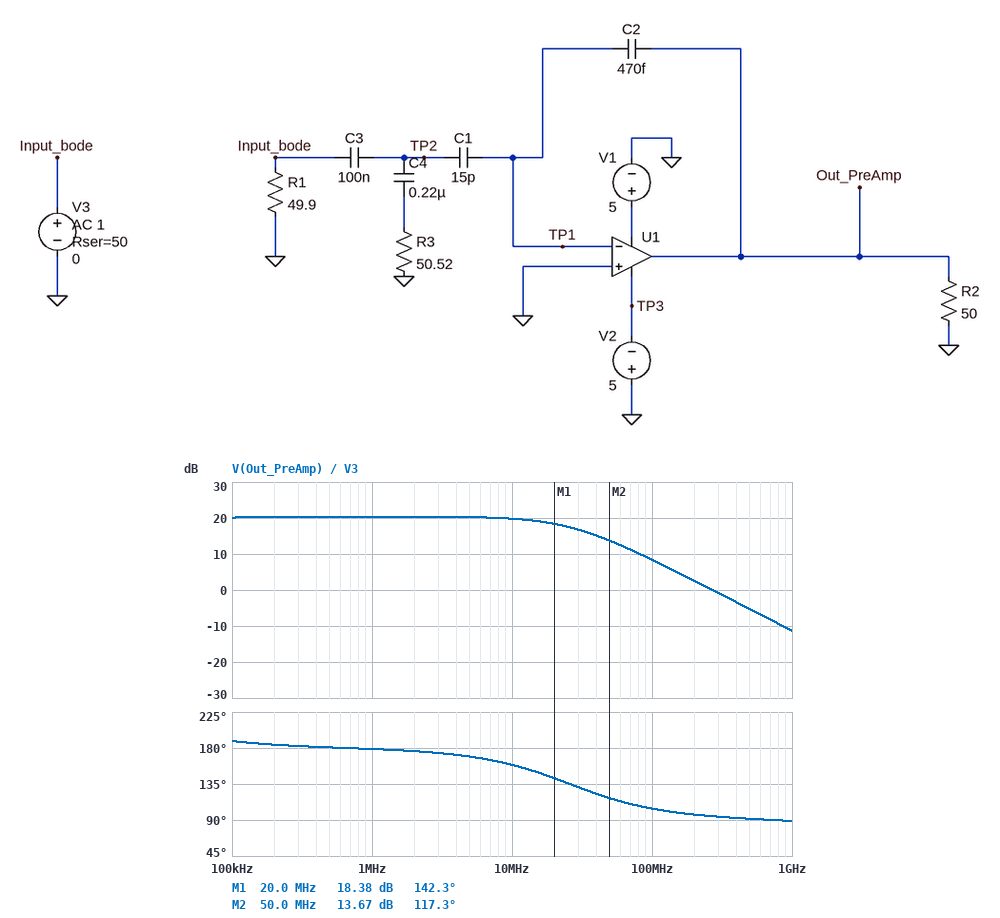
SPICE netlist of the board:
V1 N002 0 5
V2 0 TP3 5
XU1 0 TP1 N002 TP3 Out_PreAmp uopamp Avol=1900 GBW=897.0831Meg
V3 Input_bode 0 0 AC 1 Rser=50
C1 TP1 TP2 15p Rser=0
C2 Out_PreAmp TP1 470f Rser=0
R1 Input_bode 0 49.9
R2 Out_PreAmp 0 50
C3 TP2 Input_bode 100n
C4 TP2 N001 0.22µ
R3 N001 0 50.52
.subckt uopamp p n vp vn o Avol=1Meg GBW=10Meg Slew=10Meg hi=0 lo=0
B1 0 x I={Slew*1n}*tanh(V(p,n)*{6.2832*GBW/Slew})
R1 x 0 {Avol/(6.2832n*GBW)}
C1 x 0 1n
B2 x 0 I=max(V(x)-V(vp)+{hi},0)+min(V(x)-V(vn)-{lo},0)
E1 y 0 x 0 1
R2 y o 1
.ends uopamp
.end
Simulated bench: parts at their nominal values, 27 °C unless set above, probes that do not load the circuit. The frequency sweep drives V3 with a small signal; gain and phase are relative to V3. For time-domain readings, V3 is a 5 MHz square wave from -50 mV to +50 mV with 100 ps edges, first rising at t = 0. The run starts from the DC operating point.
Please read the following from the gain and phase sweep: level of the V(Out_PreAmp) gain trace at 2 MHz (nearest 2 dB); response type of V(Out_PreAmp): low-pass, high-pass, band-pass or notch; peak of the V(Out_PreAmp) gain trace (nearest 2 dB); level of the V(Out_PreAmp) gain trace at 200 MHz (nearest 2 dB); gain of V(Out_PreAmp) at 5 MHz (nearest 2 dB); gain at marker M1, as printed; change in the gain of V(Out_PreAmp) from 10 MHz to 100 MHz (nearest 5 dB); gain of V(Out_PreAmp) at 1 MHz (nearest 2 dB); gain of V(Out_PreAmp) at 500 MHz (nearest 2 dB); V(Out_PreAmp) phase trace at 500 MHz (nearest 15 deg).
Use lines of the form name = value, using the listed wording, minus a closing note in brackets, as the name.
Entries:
level of the V(Out_PreAmp) gain trace at 2 MHz = 20 dB
response type of V(Out_PreAmp): low-pass, high-pass, band-pass or notch = low-pass
peak of the V(Out_PreAmp) gain trace = 20 dB
level of the V(Out_PreAmp) gain trace at 200 MHz = 2 dB
gain of V(Out_PreAmp) at 5 MHz = 20 dB
gain at marker M1, as printed = 18.38 dB
change in the gain of V(Out_PreAmp) from 10 MHz to 100 MHz = -10 dB
gain of V(Out_PreAmp) at 1 MHz = 20 dB
gain of V(Out_PreAmp) at 500 MHz = -6 dB
V(Out_PreAmp) phase trace at 500 MHz = 90 deg
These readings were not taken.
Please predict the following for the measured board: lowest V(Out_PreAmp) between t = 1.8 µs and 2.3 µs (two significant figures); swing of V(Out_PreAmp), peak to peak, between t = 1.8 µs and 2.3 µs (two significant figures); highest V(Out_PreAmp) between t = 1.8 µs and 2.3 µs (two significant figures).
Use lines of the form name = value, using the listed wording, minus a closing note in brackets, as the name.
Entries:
lowest V(Out_PreAmp) between t = 1.8 µs and 2.3 µs = -790 mV
swing of V(Out_PreAmp), peak to peak, between t = 1.8 µs and 2.3 µs = 880 mV
highest V(Out_PreAmp) between t = 1.8 µs and 2.3 µs = 94 mV
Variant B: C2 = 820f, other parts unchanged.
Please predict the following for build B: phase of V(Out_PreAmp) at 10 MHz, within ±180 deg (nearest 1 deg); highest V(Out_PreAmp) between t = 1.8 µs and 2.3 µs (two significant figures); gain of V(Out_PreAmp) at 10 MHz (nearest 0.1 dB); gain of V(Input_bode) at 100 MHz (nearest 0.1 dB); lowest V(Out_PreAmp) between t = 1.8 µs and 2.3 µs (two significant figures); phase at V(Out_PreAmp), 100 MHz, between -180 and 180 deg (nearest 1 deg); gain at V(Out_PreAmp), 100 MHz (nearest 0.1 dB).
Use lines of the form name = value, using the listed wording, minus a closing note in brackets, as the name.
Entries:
phase of V(Out_PreAmp) at 10 MHz, within ±180 deg = 167 deg
highest V(Out_PreAmp) between t = 1.8 µs and 2.3 µs = 55 mV
gain of V(Out_PreAmp) at 10 MHz = 15.4 dB
gain of V(Input_bode) at 100 MHz = -10.0 dB
lowest V(Out_PreAmp) between t = 1.8 µs and 2.3 µs = -550 mV
phase at V(Out_PreAmp), 100 MHz, between -180 and 180 deg = 113 deg
gain at V(Out_PreAmp), 100 MHz = 7.6 dB
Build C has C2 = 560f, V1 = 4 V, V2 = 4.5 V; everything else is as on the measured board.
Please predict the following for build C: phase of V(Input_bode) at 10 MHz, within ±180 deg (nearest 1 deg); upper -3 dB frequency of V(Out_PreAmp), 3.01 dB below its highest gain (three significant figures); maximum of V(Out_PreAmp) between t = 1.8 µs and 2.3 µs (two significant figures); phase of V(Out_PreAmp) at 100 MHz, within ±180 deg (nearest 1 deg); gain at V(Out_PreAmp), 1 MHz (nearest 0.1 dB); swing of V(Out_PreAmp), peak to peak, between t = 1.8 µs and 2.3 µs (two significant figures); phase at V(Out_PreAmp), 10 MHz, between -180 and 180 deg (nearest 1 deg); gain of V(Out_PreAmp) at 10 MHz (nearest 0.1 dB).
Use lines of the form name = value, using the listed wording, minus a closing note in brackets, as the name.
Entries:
phase of V(Input_bode) at 10 MHz, within ±180 deg = -1 deg
upper -3 dB frequency of V(Out_PreAmp), 3.01 dB below its highest gain = 30.7 MHz
maximum of V(Out_PreAmp) between t = 1.8 µs and 2.3 µs = 80 mV
phase of V(Out_PreAmp) at 100 MHz, within ±180 deg = 107 deg
gain at V(Out_PreAmp), 1 MHz = 18.9 dB
swing of V(Out_PreAmp), peak to peak, between t = 1.8 µs and 2.3 µs = 860 mV
phase at V(Out_PreAmp), 10 MHz, between -180 and 180 deg = 162 deg
gain of V(Out_PreAmp) at 10 MHz = 18.5 dB
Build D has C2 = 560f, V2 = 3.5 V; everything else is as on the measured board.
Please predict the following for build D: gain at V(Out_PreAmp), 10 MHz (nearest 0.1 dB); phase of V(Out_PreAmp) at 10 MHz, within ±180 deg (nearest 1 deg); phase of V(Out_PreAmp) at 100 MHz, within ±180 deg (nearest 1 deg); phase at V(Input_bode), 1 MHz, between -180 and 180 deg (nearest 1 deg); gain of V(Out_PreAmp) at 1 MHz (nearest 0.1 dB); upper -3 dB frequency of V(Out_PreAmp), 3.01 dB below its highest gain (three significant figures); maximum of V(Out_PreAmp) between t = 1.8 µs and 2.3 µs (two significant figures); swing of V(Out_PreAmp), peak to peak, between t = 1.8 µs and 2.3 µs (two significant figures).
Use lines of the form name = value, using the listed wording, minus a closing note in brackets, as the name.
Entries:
gain at V(Out_PreAmp), 10 MHz = 18.5 dB
phase of V(Out_PreAmp) at 10 MHz, within ±180 deg = 162 deg
phase of V(Out_PreAmp) at 100 MHz, within ±180 deg = 107 deg
phase at V(Input_bode), 1 MHz, between -180 and 180 deg = -1 deg
gain of V(Out_PreAmp) at 1 MHz = 18.9 dB
upper -3 dB frequency of V(Out_PreAmp), 3.01 dB below its highest gain = 30.7 MHz
maximum of V(Out_PreAmp) between t = 1.8 µs and 2.3 µs = 80 mV
swing of V(Out_PreAmp), peak to peak, between t = 1.8 µs and 2.3 µs = 860 mV
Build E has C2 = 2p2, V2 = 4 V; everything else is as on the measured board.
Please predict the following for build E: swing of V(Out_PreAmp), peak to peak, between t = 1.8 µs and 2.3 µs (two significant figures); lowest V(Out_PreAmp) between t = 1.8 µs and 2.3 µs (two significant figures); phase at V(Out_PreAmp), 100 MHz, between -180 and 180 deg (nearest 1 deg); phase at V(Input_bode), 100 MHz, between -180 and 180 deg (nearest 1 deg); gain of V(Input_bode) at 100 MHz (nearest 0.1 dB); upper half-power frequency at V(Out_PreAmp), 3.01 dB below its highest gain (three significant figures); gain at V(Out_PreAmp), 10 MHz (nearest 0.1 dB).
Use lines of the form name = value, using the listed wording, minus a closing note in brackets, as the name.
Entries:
swing of V(Out_PreAmp), peak to peak, between t = 1.8 µs and 2.3 µs = 230 mV
lowest V(Out_PreAmp) between t = 1.8 µs and 2.3 µs = -210 mV
phase at V(Out_PreAmp), 100 MHz, between -180 and 180 deg = 133 deg
phase at V(Input_bode), 100 MHz, between -180 and 180 deg = -5 deg
gain of V(Input_bode) at 100 MHz = -10.1 dB
upper half-power frequency at V(Out_PreAmp), 3.01 dB below its highest gain = 97.7 MHz
gain at V(Out_PreAmp), 10 MHz = 7.1 dB
